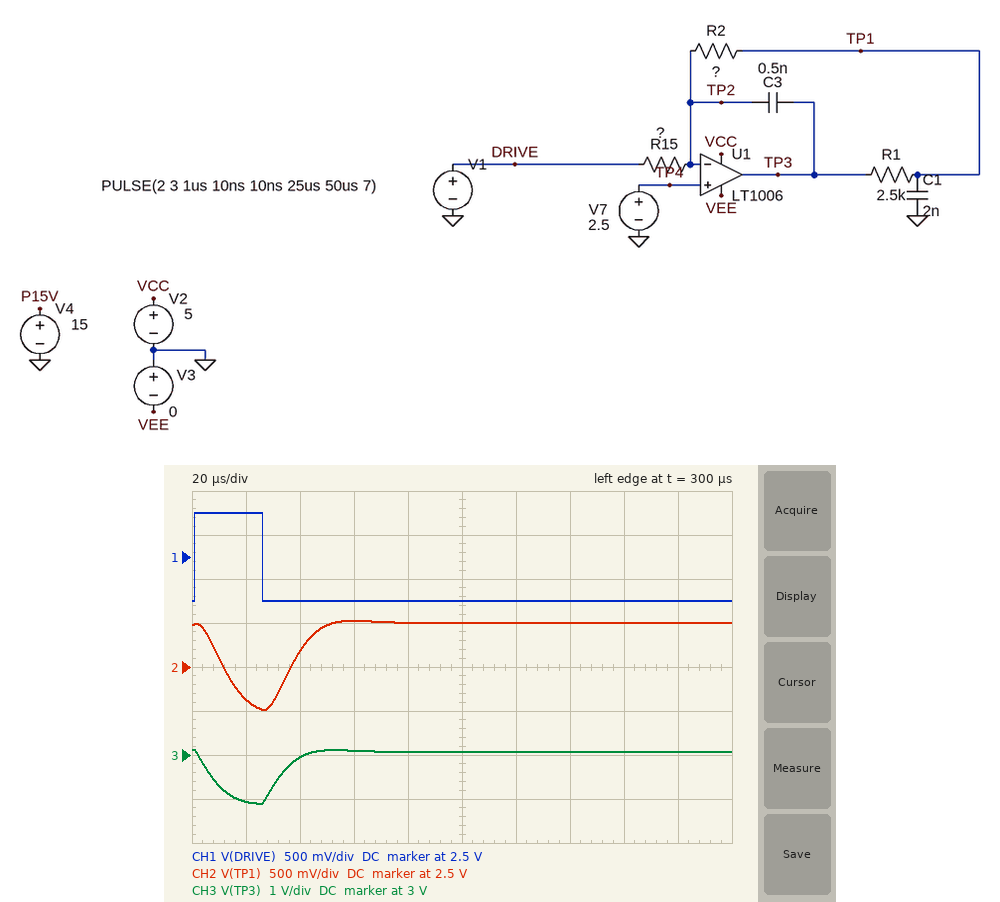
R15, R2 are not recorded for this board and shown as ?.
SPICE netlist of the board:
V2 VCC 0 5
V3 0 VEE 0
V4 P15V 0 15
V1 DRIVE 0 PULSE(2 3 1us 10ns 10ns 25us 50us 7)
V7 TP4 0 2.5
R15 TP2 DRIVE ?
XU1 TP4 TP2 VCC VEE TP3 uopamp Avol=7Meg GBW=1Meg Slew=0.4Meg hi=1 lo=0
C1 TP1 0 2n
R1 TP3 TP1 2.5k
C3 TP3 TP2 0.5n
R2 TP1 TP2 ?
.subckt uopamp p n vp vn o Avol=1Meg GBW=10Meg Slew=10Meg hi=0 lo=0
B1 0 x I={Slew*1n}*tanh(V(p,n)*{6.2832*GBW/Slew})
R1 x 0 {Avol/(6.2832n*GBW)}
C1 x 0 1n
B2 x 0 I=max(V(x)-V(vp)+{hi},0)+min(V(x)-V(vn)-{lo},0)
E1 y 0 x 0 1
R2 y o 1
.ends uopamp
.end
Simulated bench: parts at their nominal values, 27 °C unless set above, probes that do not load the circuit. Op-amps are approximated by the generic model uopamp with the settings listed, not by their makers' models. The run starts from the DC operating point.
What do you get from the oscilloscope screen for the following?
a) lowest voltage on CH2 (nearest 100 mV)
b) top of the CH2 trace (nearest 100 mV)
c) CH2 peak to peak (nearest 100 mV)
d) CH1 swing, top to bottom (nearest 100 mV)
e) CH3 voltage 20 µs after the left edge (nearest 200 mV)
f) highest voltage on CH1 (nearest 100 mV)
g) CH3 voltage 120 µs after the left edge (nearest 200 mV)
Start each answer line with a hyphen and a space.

- 2.0 V
- 3.0 V
- 1.0 V
- 1.0 V
- 2.0 V
- 3.0 V
- 3.0 V
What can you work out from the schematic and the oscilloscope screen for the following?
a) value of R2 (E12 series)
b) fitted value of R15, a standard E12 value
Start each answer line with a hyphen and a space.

- 18 kΩ
- 18 kΩ
